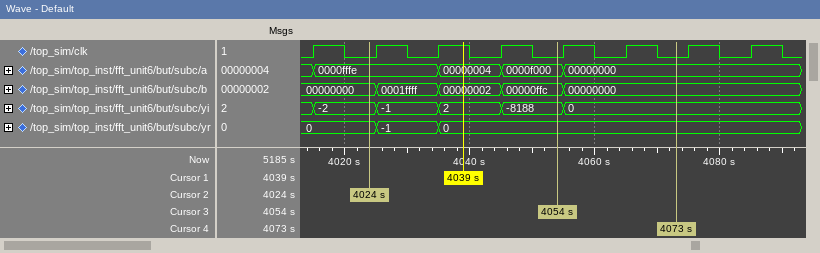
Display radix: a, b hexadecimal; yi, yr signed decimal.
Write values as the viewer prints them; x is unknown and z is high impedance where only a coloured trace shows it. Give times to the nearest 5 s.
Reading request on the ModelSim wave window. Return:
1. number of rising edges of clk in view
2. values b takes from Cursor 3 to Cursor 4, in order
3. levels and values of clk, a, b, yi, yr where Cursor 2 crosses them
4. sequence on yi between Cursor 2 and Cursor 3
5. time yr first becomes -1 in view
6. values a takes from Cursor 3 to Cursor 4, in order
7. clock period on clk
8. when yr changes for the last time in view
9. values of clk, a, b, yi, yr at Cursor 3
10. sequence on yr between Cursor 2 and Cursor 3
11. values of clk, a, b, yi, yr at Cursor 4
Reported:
8
00000ffc, 00000000
clk=0, a=0000fffe, b=00000000, yi=-2, yr=0
-2, -1, 2, -8188
4025 s
0000f000, 00000000
10 s
4035 s
clk=0, a=0000f000, b=00000ffc, yi=-8188, yr=0
0, -1, 0
clk=0, a=00000000, b=00000000, yi=0, yr=0
